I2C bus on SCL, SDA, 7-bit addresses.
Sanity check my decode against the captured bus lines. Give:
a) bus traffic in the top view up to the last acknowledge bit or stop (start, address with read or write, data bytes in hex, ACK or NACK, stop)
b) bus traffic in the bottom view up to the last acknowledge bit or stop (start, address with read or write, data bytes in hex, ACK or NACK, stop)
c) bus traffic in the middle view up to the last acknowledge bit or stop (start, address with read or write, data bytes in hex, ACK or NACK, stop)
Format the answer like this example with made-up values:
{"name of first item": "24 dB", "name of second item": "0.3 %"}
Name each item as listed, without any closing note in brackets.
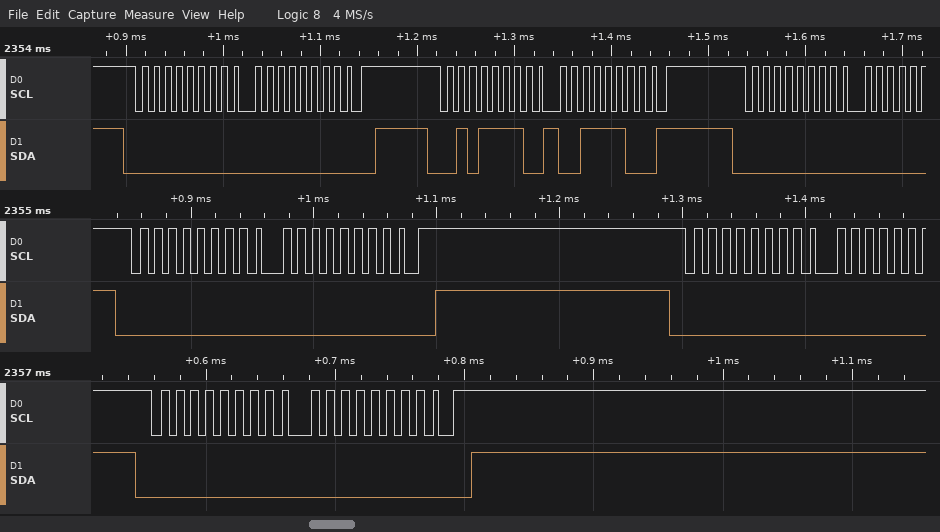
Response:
{"bus traffic in the top view up to the last acknowledge bit or stop": "start, address 00 write ACK, 00 ACK, stop, start, address 2F write ACK, 3C ACK, repeated start, address 00 write ACK", "bus traffic in the bottom view up to the last acknowledge bit or stop": "start, address 00 write ACK, 00 ACK, stop", "bus traffic in the middle view up to the last acknowledge bit or stop": "start, address 00 write ACK, 00 ACK, stop, start, address 00 write ACK"}
